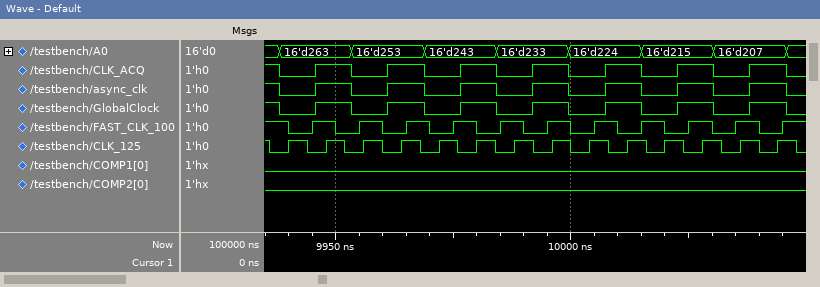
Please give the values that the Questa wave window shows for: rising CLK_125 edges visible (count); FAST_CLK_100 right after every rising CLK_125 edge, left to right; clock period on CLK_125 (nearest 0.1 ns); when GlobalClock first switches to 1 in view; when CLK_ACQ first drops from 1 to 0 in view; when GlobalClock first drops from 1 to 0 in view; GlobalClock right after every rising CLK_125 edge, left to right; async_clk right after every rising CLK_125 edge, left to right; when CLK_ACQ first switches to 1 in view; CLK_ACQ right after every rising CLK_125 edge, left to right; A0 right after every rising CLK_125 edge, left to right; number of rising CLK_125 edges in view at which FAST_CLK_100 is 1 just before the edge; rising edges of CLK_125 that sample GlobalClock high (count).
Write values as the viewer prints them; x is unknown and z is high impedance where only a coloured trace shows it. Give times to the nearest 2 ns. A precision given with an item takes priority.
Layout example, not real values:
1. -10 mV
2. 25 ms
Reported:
1. 14
2. 0 1 1 0 0 0 1 1 0 0 0 1 1 0
3. 8 ns
4. 9946 ns
5. 9938 ns
6. 9938 ns
7. 0 1 0 1 0 1 0 1 0 1 0 1 0 1
8. 0 1 0 1 0 1 0 1 0 1 0 1 0 1
9. 9946 ns
10. 0 1 0 1 0 1 0 1 0 1 0 1 0 1
11. 16'd263, 16'd263, 16'd253, 16'd253, 16'd243, 16'd243, 16'd233, 16'd233, 16'd224, 16'd224, 16'd215, 16'd215, 16'd207, 16'd207
12. 9
13. 7
